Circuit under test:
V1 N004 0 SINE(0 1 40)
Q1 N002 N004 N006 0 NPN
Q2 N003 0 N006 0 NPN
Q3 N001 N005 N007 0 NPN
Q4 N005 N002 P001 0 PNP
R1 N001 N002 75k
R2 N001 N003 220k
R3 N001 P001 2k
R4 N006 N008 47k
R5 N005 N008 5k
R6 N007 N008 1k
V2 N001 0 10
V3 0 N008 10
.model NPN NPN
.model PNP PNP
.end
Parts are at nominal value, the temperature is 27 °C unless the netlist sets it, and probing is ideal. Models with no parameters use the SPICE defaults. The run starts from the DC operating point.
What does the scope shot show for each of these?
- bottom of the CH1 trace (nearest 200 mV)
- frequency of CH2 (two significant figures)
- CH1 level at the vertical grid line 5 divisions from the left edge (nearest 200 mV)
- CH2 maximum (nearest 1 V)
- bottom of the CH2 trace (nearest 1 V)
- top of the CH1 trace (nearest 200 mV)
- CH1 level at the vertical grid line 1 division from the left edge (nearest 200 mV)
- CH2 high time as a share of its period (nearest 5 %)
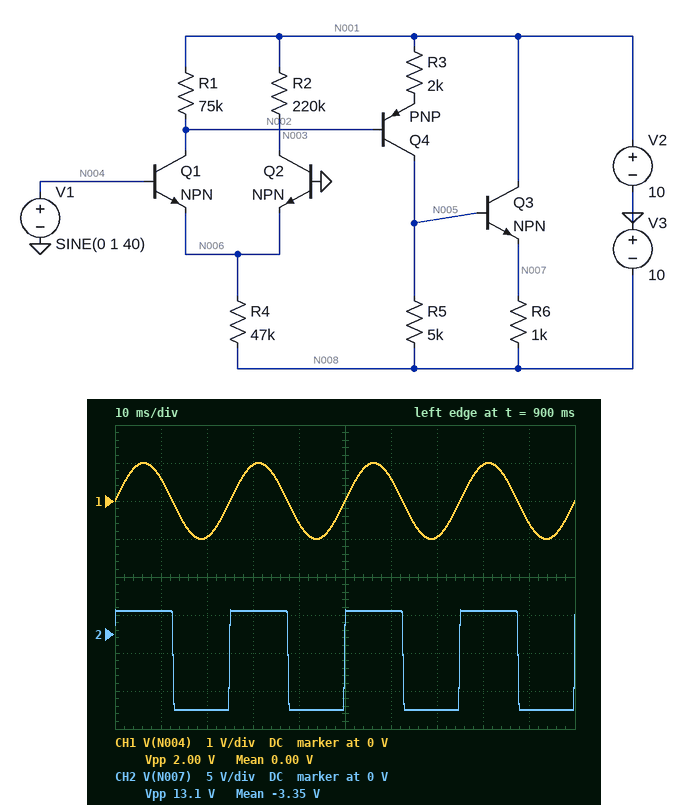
-1.0 V
40 Hz
0 V
3 V
-10 V
1.0 V
600 mV
50 %
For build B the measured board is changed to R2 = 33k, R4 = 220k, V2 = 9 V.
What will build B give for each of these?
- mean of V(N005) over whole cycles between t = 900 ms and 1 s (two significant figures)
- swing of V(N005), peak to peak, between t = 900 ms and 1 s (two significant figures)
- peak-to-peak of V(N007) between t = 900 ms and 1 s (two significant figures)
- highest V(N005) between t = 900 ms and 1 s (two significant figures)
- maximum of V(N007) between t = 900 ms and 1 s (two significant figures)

-7.8 V
4.7 V
3.9 V
-5.3 V
-6.1 V
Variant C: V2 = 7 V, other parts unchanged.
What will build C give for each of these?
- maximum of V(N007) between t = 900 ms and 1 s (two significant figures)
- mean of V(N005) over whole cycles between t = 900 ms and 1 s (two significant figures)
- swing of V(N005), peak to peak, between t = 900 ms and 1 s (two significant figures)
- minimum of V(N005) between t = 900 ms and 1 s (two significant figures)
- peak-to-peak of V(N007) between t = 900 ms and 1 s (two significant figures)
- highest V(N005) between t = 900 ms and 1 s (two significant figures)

1.0 V
-4.0 V
12 V
-10 V
11 V
1.8 V
